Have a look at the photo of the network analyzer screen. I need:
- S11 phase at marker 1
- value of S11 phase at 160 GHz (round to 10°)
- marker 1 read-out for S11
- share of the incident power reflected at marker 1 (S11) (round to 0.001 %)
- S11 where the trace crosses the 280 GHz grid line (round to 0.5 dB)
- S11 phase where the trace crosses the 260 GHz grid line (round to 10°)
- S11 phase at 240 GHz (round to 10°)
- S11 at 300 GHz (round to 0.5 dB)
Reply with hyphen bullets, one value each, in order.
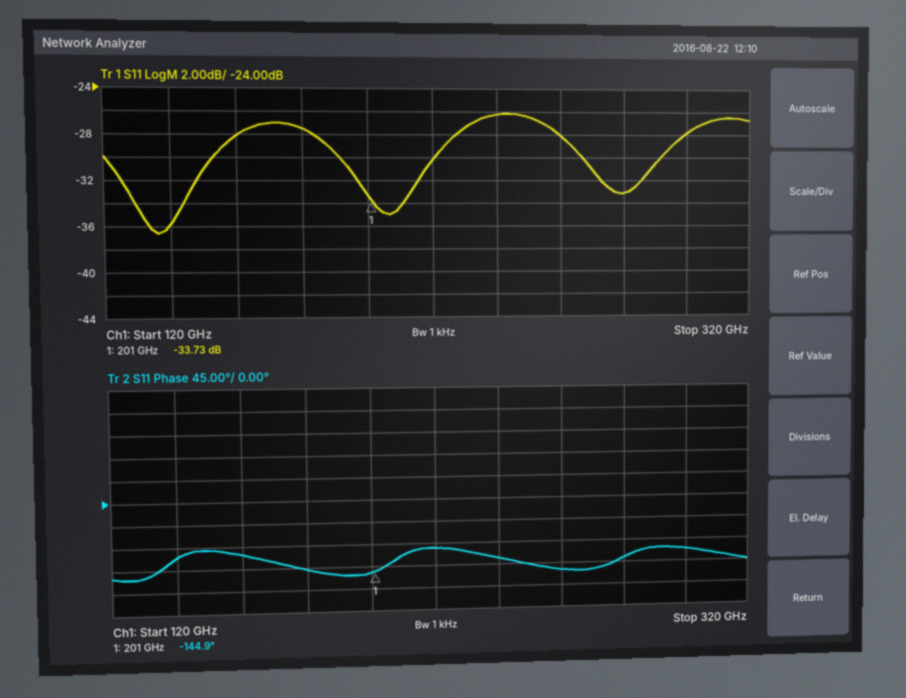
- -144.9°
- -110°
- -33.73 dB
- 0.042 %
- -33.0 dB
- -150°
- -120°
- -28.0 dB
